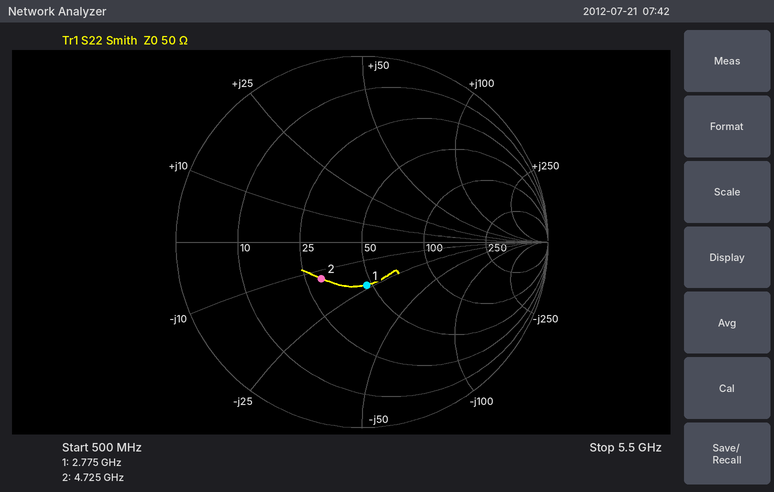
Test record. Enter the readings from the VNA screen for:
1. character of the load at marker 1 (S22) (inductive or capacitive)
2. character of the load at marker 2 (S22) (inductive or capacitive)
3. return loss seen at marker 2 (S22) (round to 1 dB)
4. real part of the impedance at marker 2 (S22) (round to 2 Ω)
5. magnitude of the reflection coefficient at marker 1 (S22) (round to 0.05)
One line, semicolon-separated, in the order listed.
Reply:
capacitive; capacitive; 11 dB; 30 Ω; 0.25
